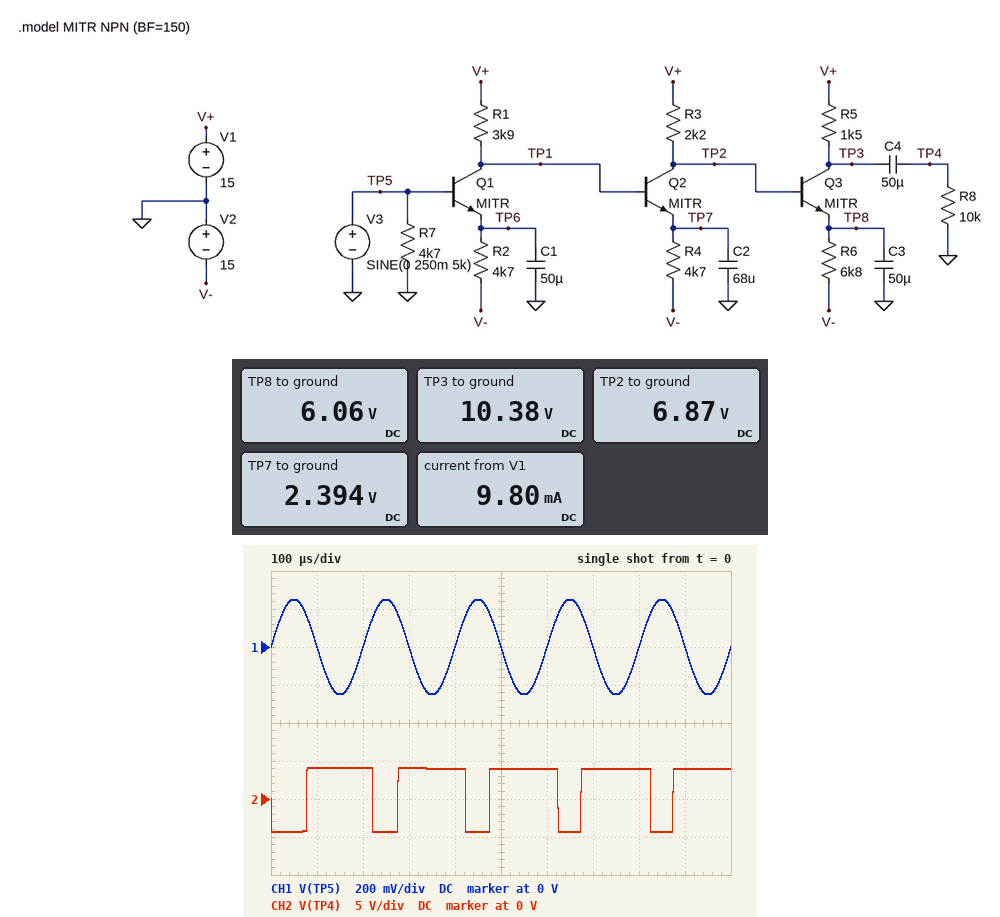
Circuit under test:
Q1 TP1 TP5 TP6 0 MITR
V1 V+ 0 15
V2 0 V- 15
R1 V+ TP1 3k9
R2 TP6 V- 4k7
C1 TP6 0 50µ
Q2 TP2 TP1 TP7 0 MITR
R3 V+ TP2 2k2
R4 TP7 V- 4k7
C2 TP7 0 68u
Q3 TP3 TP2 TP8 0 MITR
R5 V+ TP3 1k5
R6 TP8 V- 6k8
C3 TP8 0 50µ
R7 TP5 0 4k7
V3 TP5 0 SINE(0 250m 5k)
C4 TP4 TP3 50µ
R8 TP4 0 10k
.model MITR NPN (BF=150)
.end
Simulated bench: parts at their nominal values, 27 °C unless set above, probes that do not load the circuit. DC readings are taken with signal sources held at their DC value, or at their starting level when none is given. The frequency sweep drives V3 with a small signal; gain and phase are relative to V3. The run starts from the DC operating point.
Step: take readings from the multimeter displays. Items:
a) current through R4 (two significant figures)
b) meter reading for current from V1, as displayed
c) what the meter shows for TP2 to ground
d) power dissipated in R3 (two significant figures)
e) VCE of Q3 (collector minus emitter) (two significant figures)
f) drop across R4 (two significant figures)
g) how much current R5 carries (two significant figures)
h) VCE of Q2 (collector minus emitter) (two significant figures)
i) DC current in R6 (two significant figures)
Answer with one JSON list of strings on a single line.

["3.7 mA", "9.80 mA", "6.87 V", "30 mW", "4.3 V", "17 V", "3.1 mA", "4.5 V", "3.1 mA"]
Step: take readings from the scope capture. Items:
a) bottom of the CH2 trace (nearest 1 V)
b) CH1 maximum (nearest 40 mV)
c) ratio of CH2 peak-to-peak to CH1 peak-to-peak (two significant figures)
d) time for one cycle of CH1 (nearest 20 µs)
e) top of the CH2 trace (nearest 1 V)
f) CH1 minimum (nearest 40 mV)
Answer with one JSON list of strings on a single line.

["-4 V", "240 mV", "17", "200 µs", "4 V", "-240 mV"]
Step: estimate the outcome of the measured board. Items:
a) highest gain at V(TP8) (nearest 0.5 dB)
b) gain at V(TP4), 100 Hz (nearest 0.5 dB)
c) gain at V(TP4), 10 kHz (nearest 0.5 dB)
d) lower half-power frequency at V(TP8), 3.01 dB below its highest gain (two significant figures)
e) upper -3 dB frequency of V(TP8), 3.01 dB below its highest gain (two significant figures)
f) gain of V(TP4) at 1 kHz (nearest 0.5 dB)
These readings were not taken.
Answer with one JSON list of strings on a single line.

["78.0 dB", "106.5 dB", "124.5 dB", "110 Hz", "630 Hz", "124.0 dB"]
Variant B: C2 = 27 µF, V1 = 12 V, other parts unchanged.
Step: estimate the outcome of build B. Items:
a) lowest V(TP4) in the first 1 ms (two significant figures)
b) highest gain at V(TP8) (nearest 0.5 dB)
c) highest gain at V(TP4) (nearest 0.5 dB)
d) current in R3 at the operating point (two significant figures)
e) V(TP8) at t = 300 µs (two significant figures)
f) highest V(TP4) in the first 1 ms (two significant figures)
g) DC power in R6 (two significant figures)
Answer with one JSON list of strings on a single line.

["-3.3 V", "76.0 dB", "124.0 dB", "3.1 mA", "4.5 V", "3.7 V", "56 mW"]
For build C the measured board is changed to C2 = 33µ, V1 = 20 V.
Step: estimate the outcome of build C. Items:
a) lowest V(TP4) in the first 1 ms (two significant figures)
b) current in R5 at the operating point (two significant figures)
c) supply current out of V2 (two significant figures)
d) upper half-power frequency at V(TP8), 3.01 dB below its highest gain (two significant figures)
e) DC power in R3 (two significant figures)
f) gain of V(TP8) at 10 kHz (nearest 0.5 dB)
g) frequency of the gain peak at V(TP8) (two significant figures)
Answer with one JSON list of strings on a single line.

["-6.0 V", "3.5 mA", "11 mA", "720 Hz", "50 mW", "53.0 dB", "300 Hz"]
